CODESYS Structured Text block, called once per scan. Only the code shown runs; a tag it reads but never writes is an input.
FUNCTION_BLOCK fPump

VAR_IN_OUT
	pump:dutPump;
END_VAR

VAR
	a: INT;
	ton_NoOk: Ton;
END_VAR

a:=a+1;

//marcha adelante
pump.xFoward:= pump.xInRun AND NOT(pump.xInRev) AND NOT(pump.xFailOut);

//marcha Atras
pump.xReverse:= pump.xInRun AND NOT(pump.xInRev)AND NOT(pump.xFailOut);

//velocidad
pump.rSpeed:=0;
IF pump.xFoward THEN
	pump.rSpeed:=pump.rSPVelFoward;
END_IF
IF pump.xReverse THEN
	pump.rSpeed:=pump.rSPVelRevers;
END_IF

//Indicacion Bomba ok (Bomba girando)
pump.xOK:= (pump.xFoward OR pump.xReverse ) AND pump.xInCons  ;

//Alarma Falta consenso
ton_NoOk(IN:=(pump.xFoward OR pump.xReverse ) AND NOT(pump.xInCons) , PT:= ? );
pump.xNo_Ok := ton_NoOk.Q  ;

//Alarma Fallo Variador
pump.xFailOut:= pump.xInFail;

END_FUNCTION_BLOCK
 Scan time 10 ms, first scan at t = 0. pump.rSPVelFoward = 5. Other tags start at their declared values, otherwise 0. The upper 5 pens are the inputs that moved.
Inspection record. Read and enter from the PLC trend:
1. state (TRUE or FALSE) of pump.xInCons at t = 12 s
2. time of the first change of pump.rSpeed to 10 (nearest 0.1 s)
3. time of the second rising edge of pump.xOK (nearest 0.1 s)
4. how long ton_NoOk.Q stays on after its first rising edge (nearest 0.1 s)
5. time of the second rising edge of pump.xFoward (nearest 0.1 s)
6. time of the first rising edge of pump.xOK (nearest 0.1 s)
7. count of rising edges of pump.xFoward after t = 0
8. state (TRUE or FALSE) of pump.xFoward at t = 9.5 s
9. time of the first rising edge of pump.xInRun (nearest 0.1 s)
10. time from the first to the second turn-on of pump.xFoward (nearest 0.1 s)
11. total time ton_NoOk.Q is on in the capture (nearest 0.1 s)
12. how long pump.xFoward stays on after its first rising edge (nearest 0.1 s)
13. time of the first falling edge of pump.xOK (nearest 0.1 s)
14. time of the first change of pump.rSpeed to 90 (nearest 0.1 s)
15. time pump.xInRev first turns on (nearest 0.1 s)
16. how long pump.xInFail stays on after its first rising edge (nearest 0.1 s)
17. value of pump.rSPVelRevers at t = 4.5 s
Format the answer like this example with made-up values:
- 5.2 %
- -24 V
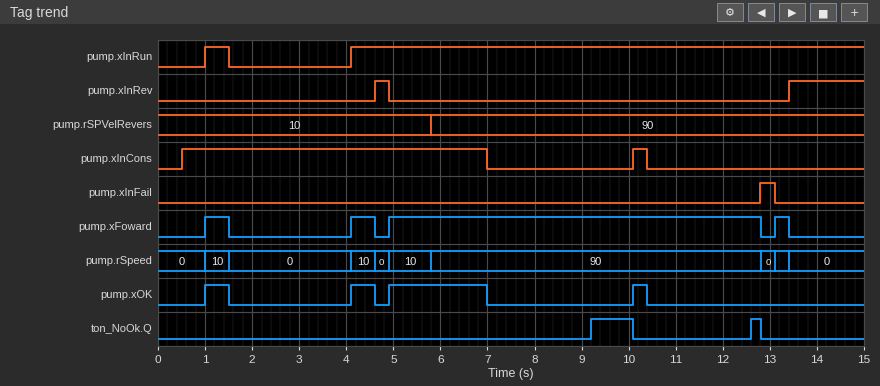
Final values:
- FALSE
- 1.0 s
- 4.1 s
- 0.9 s
- 4.1 s
- 1.0 s
- 4
- TRUE
- 1.0 s
- 3.1 s
- 1.1 s
- 0.5 s
- 1.5 s
- 5.8 s
- 4.6 s
- 0.3 s
- 10
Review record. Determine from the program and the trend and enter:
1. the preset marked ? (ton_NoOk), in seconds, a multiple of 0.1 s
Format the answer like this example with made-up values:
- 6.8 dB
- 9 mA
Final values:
- 2.2 s
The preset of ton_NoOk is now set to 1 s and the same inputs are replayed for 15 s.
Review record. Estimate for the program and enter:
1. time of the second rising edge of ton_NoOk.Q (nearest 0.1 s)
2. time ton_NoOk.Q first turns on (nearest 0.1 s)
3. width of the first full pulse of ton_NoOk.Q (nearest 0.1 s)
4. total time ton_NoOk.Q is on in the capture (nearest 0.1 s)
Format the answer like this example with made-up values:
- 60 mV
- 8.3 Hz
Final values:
- 11.4 s
- 8.0 s
- 2.1 s
- 3.5 s
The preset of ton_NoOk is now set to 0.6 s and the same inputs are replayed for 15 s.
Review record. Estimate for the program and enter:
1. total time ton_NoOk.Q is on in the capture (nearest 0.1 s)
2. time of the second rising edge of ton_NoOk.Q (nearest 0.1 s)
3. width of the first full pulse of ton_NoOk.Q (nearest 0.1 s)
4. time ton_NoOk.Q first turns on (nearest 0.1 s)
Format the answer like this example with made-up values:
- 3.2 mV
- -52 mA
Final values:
- 4.3 s
- 11.0 s
- 2.5 s
- 7.6 s
